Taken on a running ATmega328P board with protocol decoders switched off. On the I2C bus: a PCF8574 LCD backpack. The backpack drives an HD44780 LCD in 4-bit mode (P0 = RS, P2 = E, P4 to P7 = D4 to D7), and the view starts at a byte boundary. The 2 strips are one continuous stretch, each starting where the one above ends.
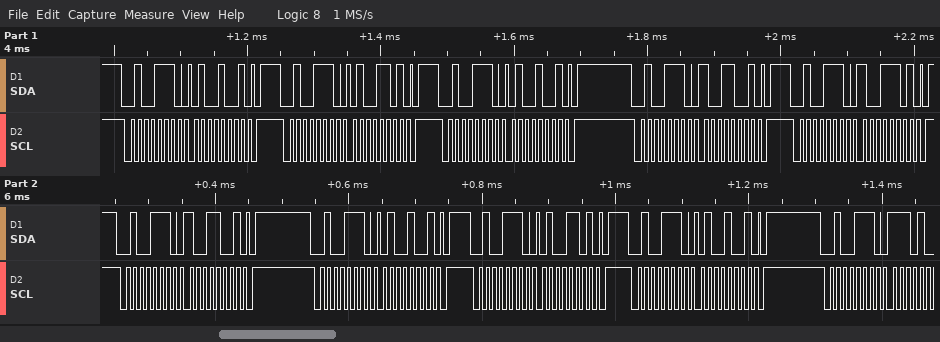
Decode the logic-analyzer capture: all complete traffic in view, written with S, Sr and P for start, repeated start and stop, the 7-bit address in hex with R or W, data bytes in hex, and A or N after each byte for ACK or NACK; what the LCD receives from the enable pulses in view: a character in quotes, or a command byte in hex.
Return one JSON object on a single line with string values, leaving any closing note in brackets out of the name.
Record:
{"all complete traffic in view, written with S, Sr and P for start, repeated start and stop, the 7-bit address in hex with R or W, data bytes in hex, and A or N after each byte for ACK or NACK": "S 27W A 49 A P S 27W A 4D A P S 27W A 49 A P S 27W A 99 A P S 27W A 9D A P S 27W A 99 A P S 27W A 49 A P S 27W A 4D A P S 27W A 49 A P S 27W A", "what the LCD receives from the enable pulses in view: a character in quotes, or a command byte in hex": "'I'"}
